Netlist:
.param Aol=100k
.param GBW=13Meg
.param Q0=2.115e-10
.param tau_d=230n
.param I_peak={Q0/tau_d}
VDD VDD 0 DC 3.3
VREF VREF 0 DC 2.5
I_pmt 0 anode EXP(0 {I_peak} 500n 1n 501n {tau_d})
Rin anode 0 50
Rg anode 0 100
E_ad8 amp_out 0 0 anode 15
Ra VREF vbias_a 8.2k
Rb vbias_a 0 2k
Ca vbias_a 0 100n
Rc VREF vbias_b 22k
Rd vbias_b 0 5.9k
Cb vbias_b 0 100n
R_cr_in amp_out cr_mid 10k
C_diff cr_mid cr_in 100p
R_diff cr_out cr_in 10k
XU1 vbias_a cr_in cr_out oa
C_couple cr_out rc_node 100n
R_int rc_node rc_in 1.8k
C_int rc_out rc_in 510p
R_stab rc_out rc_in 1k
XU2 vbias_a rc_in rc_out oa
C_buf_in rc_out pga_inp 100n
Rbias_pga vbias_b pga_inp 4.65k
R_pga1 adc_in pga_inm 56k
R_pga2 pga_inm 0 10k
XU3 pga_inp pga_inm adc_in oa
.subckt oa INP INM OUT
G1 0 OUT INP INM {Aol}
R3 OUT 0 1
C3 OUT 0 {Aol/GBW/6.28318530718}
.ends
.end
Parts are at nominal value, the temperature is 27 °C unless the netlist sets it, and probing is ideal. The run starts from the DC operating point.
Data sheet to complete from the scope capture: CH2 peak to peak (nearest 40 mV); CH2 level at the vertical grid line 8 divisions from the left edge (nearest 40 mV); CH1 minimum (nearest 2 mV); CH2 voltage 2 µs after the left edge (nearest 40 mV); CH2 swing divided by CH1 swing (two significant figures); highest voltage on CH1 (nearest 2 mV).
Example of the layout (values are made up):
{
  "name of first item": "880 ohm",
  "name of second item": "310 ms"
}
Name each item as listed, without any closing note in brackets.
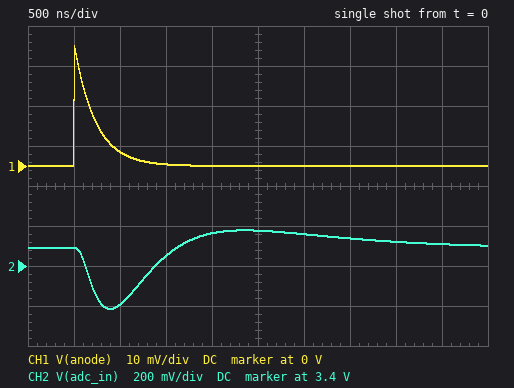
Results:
{
  "CH2 peak to peak": "400 mV",
  "CH2 level at the vertical grid line 8 divisions from the left edge": "3.52 V",
  "CH1 minimum": "0 V",
  "CH2 voltage 2 µs after the left edge": "3.56 V",
  "CH2 swing divided by CH1 swing": "13",
  "highest voltage on CH1": "30 mV"
}
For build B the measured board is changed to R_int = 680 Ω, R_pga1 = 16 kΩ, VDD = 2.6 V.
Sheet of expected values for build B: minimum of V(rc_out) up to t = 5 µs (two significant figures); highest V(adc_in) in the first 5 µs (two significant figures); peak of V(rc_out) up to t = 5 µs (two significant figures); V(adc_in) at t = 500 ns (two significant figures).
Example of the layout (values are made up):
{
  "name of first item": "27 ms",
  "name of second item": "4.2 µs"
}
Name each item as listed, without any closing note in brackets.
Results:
{
  "minimum of V(rc_out) up to t = 5 µs": "360 mV",
  "highest V(adc_in) in the first 5 µs": "1.5 V",
  "peak of V(rc_out) up to t = 5 µs": "530 mV",
  "V(adc_in) at t = 500 ns": "1.4 V"
}
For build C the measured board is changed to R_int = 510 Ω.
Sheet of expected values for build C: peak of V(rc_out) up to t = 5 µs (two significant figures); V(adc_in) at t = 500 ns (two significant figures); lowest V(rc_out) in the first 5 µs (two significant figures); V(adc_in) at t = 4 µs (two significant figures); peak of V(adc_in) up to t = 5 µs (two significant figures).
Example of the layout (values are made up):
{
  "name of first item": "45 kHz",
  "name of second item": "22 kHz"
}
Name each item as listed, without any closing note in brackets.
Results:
{
  "peak of V(rc_out) up to t = 5 µs": "540 mV",
  "V(adc_in) at t = 500 ns": "3.5 V",
  "lowest V(rc_out) in the first 5 µs": "320 mV",
  "V(adc_in) at t = 4 µs": "3.6 V",
  "peak of V(adc_in) up to t = 5 µs": "3.8 V"
}
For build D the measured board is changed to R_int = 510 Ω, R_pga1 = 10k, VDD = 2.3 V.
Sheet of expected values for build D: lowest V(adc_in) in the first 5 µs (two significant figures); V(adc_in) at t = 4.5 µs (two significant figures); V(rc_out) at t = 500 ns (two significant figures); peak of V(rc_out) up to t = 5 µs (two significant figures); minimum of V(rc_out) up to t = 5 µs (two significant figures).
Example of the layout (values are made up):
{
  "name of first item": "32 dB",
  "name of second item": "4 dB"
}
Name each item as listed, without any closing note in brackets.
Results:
{
  "lowest V(adc_in) in the first 5 µs": "720 mV",
  "V(adc_in) at t = 4.5 µs": "1.1 V",
  "V(rc_out) at t = 500 ns": "490 mV",
  "peak of V(rc_out) up to t = 5 µs": "540 mV",
  "minimum of V(rc_out) up to t = 5 µs": "320 mV"
}
